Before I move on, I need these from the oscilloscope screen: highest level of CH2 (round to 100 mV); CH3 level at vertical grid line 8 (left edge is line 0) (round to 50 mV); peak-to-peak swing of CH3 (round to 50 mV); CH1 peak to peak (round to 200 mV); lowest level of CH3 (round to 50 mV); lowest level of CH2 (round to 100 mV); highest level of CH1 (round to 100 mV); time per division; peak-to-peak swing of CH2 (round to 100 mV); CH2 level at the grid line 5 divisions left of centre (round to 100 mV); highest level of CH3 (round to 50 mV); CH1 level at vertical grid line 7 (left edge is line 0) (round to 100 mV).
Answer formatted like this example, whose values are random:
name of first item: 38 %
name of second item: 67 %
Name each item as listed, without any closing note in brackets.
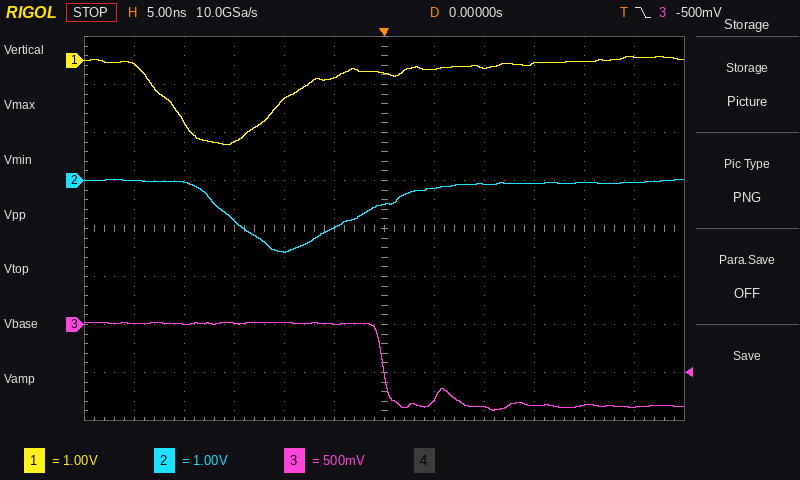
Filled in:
highest level of CH2: 0.0 V
CH3 level at vertical grid line 8 (left edge is line 0): -850 mV
peak-to-peak swing of CH3: 900 mV
CH1 peak to peak: 1.8 V
lowest level of CH3: -900 mV
lowest level of CH2: -1.5 V
highest level of CH1: 100 mV
time per division: 5 ns
peak-to-peak swing of CH2: 1.5 V
CH2 level at the grid line 5 divisions left of centre: 0.0 V
highest level of CH3: 0 mV
CH1 level at vertical grid line 7 (left edge is line 0): -200 mV
